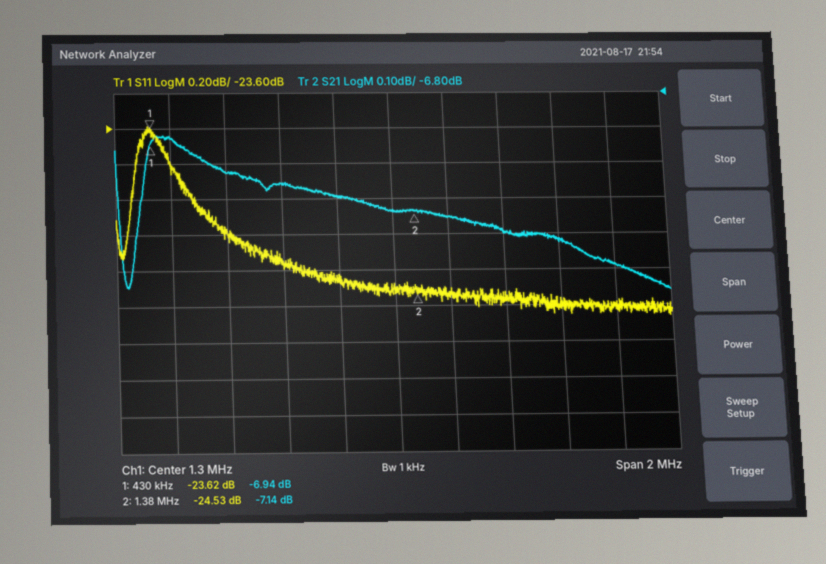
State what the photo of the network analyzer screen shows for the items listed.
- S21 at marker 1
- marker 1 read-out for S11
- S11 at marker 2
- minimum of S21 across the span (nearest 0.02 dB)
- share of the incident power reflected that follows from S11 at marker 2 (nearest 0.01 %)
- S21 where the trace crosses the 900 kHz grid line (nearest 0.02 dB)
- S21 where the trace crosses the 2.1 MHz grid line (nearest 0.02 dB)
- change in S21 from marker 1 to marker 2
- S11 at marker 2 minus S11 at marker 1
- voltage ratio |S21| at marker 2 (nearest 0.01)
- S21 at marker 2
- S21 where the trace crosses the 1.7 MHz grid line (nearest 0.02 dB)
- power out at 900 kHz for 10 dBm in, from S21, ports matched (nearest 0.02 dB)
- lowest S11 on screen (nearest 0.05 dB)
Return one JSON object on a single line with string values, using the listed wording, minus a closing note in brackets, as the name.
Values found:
{"S21 at marker 1": "-6.94 dB", "marker 1 read-out for S11": "-23.62 dB", "S11 at marker 2": "-24.53 dB", "minimum of S21 across the span": "-7.36 dB", "share of the incident power reflected that follows from S11 at marker 2": "0.35 %", "S21 where the trace crosses the 900 kHz grid line": "-7.06 dB", "S21 where the trace crosses the 2.1 MHz grid line": "-7.28 dB", "change in S21 from marker 1 to marker 2": "-0.20 dB", "S11 at marker 2 minus S11 at marker 1": "-0.91 dB", "voltage ratio |S21| at marker 2": "0.44", "S21 at marker 2": "-7.14 dB", "S21 where the trace crosses the 1.7 MHz grid line": "-7.20 dB", "power out at 900 kHz for 10 dBm in, from S21, ports matched": "2.94 dBm", "lowest S11 on screen": "-24.65 dB"}
